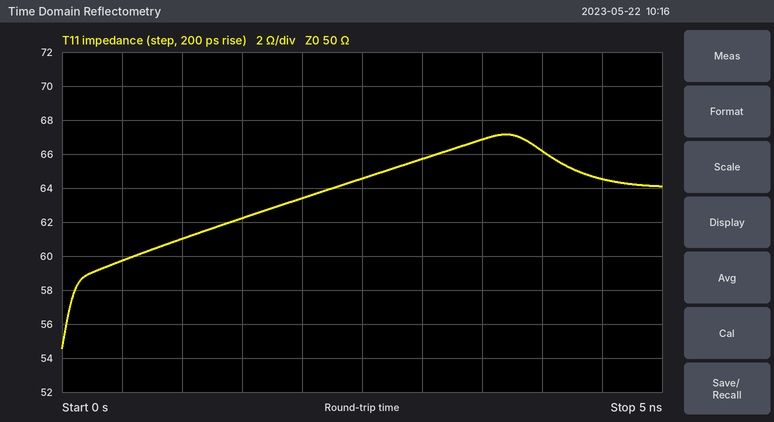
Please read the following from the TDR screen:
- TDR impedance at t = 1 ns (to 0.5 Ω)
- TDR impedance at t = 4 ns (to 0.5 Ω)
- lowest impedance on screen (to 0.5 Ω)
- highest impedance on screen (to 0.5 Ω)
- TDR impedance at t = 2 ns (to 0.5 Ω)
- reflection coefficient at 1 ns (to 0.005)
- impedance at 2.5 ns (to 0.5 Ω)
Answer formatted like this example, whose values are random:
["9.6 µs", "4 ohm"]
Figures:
["61.0 Ω", "66.0 Ω", "54.5 Ω", "67.0 Ω", "63.5 Ω", "+0.100", "64.5 Ω"]
